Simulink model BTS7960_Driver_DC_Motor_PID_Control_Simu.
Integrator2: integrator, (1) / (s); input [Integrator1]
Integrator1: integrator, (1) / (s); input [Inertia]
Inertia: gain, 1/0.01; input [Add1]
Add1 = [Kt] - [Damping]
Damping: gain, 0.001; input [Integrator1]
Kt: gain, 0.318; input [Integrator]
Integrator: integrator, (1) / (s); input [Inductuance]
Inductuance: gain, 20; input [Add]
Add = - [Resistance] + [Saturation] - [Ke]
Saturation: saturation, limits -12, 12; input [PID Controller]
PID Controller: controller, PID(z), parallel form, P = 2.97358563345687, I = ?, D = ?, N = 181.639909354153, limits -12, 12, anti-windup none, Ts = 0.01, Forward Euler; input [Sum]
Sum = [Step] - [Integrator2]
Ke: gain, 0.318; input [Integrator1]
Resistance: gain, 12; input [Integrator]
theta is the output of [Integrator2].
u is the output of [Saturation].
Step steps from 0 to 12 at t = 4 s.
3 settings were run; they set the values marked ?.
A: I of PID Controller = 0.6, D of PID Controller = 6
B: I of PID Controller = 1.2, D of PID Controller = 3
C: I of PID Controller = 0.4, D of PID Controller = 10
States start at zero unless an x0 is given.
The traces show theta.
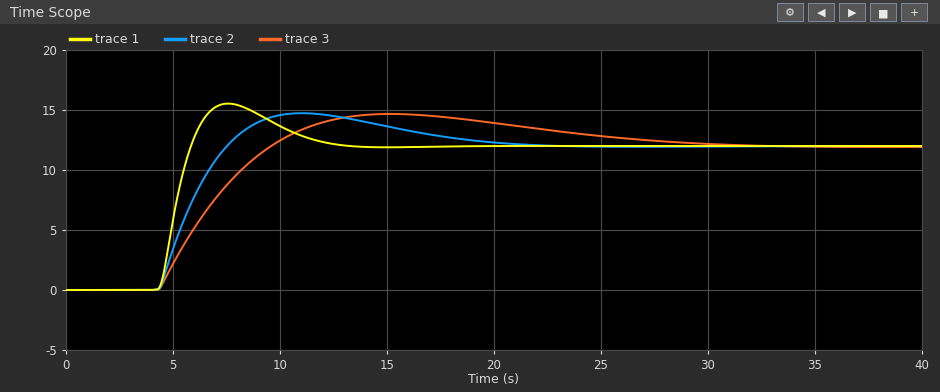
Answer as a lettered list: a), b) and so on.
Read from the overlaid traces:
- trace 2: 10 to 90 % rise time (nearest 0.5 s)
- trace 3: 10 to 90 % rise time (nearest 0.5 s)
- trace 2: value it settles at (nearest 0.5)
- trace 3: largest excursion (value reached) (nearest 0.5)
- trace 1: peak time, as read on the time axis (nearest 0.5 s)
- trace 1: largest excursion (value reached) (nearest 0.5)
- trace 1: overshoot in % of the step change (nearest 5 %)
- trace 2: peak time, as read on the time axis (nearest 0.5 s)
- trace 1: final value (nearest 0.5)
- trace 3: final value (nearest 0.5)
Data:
a) 2.5 s
b) 4.0 s
c) 12.0
d) 14.5
e) 7.5 s
f) 15.5
g) 30 %
h) 11.0 s
i) 12.0
j) 12.0
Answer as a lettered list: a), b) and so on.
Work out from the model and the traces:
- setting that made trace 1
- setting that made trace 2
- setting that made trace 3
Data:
a) B
b) A
c) C
